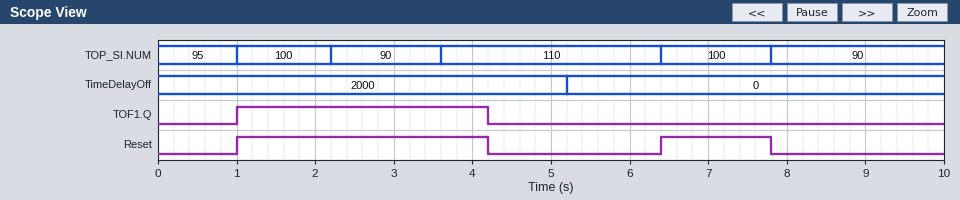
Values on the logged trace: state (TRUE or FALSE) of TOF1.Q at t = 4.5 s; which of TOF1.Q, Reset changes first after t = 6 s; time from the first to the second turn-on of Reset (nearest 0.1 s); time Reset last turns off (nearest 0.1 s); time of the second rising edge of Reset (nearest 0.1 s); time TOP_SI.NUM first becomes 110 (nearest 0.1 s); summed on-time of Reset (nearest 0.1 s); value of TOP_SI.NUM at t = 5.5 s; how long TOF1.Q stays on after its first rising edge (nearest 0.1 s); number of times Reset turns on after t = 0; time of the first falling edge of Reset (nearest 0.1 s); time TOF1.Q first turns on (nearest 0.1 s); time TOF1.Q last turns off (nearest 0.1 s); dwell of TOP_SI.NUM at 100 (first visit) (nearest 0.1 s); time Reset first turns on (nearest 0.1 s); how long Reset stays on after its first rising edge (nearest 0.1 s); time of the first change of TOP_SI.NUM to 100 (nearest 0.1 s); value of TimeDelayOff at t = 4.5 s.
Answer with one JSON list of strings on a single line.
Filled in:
["FALSE", "Reset", "5.4 s", "7.8 s", "6.4 s", "3.6 s", "4.6 s", "110", "3.2 s", "2", "4.2 s", "1.0 s", "4.2 s", "1.2 s", "1.0 s", "3.2 s", "1.0 s", "2000"]
